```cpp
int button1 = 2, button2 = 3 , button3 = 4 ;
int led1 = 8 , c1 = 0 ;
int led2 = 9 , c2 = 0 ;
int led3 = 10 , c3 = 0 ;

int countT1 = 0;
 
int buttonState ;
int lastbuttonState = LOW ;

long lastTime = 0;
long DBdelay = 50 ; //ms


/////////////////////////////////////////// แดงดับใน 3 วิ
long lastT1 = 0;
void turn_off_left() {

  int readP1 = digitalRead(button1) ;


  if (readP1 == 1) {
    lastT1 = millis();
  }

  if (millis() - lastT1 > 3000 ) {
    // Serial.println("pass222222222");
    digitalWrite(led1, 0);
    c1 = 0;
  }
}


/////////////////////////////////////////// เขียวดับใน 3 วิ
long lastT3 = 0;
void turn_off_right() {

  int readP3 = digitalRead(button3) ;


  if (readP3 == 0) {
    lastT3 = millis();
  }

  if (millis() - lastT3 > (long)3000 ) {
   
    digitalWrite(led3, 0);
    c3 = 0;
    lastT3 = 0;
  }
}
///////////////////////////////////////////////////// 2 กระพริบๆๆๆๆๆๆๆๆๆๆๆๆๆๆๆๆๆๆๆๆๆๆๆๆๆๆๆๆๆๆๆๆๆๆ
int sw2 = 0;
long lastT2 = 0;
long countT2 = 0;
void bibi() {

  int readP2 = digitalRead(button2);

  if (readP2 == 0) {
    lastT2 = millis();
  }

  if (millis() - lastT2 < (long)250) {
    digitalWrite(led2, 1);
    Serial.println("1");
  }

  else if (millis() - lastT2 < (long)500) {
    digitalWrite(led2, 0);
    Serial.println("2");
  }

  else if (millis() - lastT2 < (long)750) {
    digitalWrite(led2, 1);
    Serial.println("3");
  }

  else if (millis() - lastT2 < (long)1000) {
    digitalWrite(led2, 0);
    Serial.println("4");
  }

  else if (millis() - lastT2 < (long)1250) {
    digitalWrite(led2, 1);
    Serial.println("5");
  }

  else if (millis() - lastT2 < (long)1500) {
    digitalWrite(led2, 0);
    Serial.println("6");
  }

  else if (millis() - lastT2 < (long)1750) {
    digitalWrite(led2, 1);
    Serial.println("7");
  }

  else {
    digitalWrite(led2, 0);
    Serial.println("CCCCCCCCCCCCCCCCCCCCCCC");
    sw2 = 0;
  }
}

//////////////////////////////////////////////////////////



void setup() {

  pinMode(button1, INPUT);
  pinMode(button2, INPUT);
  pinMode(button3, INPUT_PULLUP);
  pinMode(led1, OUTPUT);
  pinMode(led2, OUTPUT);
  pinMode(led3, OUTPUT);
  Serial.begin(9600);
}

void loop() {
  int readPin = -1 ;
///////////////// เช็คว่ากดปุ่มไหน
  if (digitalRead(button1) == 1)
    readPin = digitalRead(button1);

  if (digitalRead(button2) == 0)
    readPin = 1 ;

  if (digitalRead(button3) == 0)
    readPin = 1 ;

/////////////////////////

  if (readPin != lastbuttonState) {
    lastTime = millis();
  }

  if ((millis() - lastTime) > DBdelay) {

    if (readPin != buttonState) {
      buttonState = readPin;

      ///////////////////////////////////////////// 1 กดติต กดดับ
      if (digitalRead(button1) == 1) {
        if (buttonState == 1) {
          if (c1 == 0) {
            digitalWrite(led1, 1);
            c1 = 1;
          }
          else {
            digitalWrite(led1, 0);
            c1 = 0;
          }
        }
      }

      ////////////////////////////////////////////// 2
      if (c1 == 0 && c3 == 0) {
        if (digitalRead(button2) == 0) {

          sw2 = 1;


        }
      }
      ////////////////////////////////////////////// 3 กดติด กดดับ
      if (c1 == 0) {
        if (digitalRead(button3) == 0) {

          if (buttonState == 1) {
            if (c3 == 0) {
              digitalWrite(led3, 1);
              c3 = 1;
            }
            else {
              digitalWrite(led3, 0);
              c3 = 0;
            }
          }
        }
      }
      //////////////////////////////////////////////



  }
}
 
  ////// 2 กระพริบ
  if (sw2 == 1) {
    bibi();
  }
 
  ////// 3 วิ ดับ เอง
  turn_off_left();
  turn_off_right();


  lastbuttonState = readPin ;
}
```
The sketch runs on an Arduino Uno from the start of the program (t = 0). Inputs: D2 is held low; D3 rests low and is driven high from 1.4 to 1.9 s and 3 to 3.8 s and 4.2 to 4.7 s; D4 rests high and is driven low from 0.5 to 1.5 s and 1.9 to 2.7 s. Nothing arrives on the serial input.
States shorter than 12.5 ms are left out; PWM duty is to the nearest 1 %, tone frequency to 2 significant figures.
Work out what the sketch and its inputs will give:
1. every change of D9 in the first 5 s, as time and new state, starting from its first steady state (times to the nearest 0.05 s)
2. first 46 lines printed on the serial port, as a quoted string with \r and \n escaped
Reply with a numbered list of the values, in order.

1. 0 s low; 0.05 s high; 1.65 s low; 1.9 s high; 3.25 s low; 3.5 s high; 3.75 s low; 3.8 s high; 4.45 s low; 4.7 s high
2. "1\r\n1\r\n1\r\n1\r\n1\r\n1\r\n1\r\n1\r\n1\r\n1\r\n1\r\n1\r\n1\r\n1\r\n1\r\n1\r\n1\r\n1\r\n1\r\n1\r\n1\r\n1\r\n1\r\n1\r\n1\r\n1\r\n1\r\n1\r\n1\r\n1\r\n1\r\n1\r\n1\r\n1\r\n1\r\n1\r\n1\r\n1\r\n1\r\n1\r\n1\r\n1\r\n1\r\n1\r\n1\r\n1\r\n"
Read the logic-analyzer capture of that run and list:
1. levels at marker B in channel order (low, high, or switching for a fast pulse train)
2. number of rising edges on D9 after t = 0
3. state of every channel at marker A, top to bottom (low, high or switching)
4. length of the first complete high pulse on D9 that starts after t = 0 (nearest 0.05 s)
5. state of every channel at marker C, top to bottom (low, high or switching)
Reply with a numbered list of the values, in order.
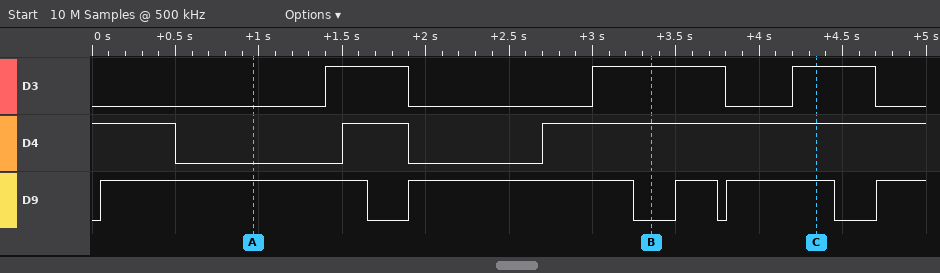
1. D3 high, D4 high, D9 low
2. 5
3. D3 low, D4 low, D9 high
4. 1.60 s
5. D3 high, D4 high, D9 high
